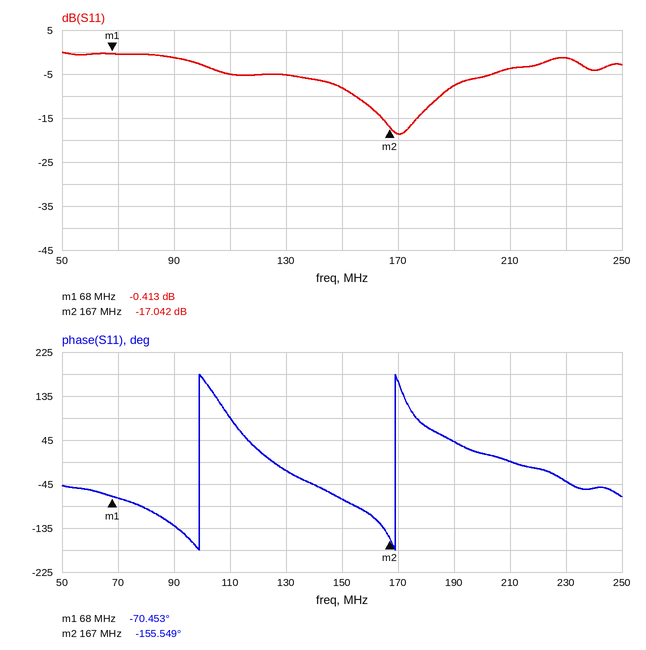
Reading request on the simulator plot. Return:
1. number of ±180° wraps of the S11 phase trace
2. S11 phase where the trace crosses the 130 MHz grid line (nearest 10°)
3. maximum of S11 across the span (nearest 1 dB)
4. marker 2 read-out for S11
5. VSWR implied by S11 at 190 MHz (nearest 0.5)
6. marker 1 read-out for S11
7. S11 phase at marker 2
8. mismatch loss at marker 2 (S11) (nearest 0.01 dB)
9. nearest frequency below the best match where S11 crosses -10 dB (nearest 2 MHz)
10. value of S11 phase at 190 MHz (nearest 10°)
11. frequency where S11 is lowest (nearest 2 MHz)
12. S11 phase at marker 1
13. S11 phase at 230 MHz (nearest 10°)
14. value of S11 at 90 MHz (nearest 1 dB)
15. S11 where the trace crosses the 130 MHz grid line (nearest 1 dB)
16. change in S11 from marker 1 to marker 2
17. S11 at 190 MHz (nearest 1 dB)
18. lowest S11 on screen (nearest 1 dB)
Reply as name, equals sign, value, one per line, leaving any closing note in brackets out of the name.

number of ±180° wraps of the S11 phase trace = 2
S11 phase where the trace crosses the 130 MHz grid line = -20°
maximum of S11 across the span = 0 dB
marker 2 read-out for S11 = -17.042 dB
VSWR implied by S11 at 190 MHz = 2.5
marker 1 read-out for S11 = -0.413 dB
S11 phase at marker 2 = -155.549°
mismatch loss at marker 2 (S11) = 0.09 dB
nearest frequency below the best match where S11 crosses -10 dB = 154 MHz
value of S11 phase at 190 MHz = 40°
frequency where S11 is lowest = 170 MHz
S11 phase at marker 1 = -70.453°
S11 phase at 230 MHz = -40°
value of S11 at 90 MHz = -1 dB
S11 where the trace crosses the 130 MHz grid line = -5 dB
change in S11 from marker 1 to marker 2 = -16.629 dB
S11 at 190 MHz = -8 dB
lowest S11 on screen = -19 dB
